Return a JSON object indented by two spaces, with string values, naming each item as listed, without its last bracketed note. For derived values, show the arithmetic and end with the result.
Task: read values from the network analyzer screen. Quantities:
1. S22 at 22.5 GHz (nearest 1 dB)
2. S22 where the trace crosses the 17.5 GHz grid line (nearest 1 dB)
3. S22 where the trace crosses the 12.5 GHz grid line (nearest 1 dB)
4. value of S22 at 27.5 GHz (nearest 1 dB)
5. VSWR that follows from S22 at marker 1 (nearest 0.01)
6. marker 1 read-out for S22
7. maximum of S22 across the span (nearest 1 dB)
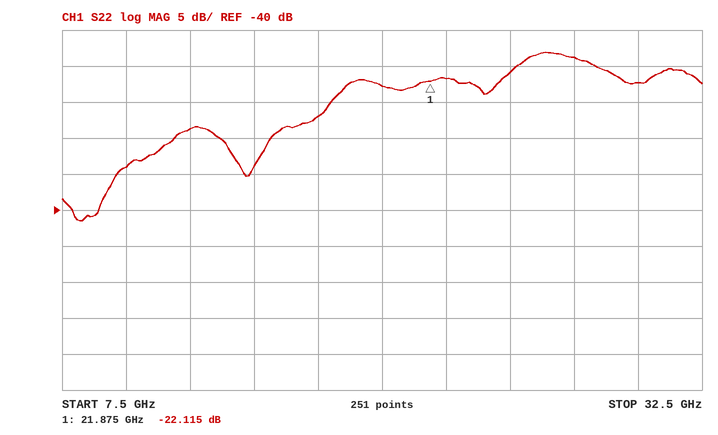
{
  "S22 at 22.5 GHz": "-22 dB",
  "S22 where the trace crosses the 17.5 GHz grid line": "-27 dB",
  "S22 where the trace crosses the 12.5 GHz grid line": "-29 dB",
  "value of S22 at 27.5 GHz": "-19 dB",
  "VSWR that follows from S22 at marker 1": "(1 + 0.0784)/(1 − 0.0784) ≈ 1.17",
  "marker 1 read-out for S22": "-22.115 dB",
  "maximum of S22 across the span": "-18 dB"
}
